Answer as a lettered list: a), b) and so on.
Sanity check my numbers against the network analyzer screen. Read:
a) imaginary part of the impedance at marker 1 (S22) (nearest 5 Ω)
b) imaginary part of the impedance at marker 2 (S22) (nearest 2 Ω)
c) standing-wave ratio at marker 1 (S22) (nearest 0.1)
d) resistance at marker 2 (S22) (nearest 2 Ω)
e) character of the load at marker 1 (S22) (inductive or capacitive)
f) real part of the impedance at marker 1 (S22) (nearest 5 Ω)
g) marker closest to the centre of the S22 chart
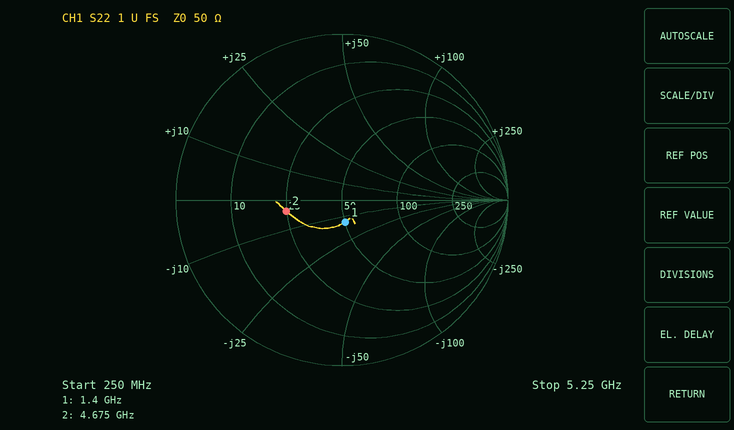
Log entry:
a) -15 Ω
b) -4 Ω
c) 1.3
d) 24 Ω
e) capacitive
f) 50 Ω
g) marker 1
